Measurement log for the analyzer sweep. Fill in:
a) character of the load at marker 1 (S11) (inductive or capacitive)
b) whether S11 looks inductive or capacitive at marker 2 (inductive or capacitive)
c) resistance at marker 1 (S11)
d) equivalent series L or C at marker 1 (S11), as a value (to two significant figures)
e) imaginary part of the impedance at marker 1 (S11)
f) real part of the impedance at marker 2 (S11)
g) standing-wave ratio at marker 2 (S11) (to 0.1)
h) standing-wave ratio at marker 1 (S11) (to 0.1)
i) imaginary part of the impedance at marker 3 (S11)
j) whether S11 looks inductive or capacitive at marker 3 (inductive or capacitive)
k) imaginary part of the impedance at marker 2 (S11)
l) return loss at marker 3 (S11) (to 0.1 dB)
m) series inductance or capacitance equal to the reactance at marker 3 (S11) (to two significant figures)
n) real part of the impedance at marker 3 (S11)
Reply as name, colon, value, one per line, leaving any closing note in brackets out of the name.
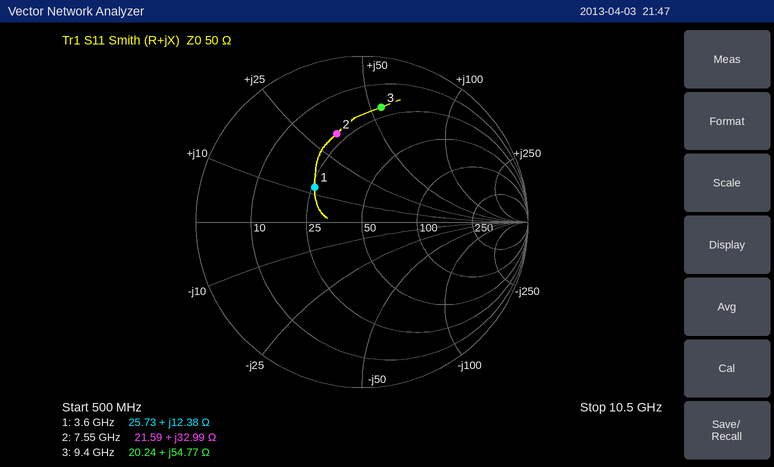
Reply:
character of the load at marker 1 (S11): inductive
whether S11 looks inductive or capacitive at marker 2: inductive
resistance at marker 1: 25.73 Ω
equivalent series L or C at marker 1 (S11), as a value: 550 pH
imaginary part of the impedance at marker 1: +12.38 Ω
real part of the impedance at marker 2: 21.59 Ω
standing-wave ratio at marker 2 (S11): 3.5
standing-wave ratio at marker 1 (S11): 2.1
imaginary part of the impedance at marker 3: +54.77 Ω
whether S11 looks inductive or capacitive at marker 3: inductive
imaginary part of the impedance at marker 2: +32.99 Ω
return loss at marker 3 (S11): 3.1 dB
series inductance or capacitance equal to the reactance at marker 3 (S11): 930 pH
real part of the impedance at marker 3: 20.24 Ω
